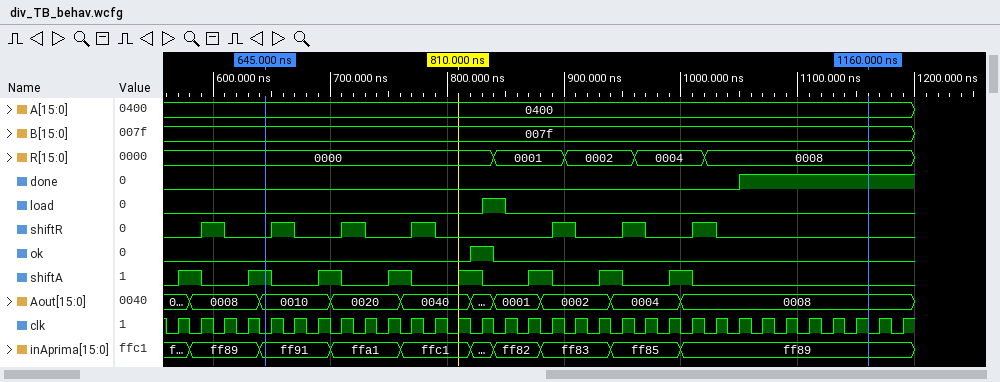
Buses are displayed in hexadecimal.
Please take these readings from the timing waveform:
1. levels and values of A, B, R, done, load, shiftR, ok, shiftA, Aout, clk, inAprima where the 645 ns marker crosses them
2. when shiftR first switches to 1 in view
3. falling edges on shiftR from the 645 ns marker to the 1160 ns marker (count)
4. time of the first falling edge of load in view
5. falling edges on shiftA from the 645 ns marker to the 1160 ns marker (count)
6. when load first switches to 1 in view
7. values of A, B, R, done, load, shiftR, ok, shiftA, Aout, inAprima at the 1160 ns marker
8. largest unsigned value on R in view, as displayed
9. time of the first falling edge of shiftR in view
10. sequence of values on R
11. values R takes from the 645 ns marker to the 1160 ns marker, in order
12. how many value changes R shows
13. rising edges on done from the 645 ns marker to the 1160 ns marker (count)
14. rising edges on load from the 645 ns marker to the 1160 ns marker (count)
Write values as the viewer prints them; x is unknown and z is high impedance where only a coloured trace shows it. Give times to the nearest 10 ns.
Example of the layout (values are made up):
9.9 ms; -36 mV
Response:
A=0400, B=007f, R=0000, done=0, load=0, shiftR=0, ok=0, shiftA=1, Aout=0010, clk=0, inAprima=ff91; 590 ns; 6; 850 ns; 7; 830 ns; A=0400, B=007f, R=0008, done=1, load=0, shiftR=0, ok=0, shiftA=0, Aout=0008, inAprima=ff89; 0008; 610 ns; 0000, 0001, 0002, 0004, 0008; 0000, 0001, 0002, 0004, 0008; 4; 1; 1
